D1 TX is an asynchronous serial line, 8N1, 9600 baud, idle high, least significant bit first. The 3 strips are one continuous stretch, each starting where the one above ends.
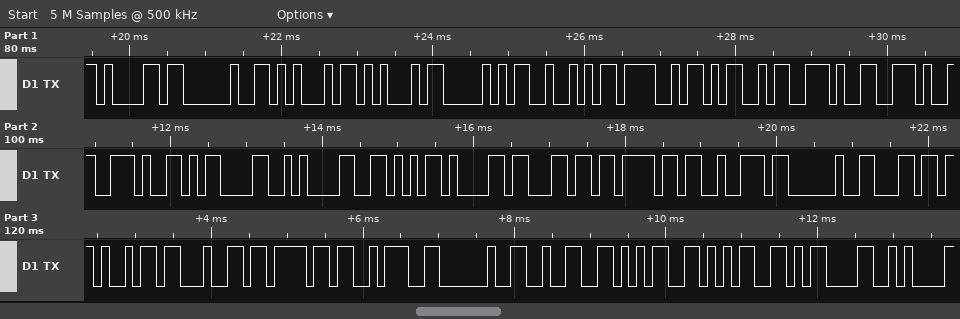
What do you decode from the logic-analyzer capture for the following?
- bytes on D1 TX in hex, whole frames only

61 20 45 45 50 52 4F 4D 2E 2E 2E 0D 0A 56 61 6C 6F 72 20 6C 69 64 6F 3A 20 32 35 35 0D 0A
